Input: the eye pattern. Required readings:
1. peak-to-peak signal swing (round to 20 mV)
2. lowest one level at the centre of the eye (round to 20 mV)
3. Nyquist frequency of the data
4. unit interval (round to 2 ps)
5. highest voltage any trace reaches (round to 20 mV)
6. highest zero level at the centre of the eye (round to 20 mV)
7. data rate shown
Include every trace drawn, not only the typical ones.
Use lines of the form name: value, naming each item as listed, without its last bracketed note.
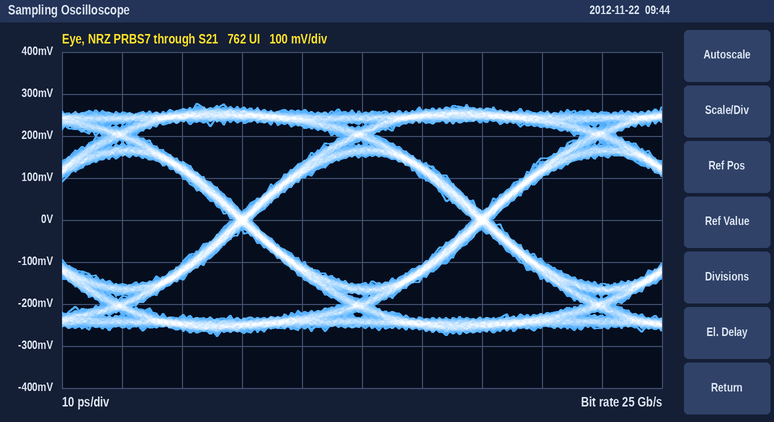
peak-to-peak signal swing: 560 mV
lowest one level at the centre of the eye: 160 mV
Nyquist frequency of the data: 12.5 GHz
unit interval: 40 ps
highest voltage any trace reaches: 280 mV
highest zero level at the centre of the eye: -160 mV
data rate shown: 25 Gb/s
